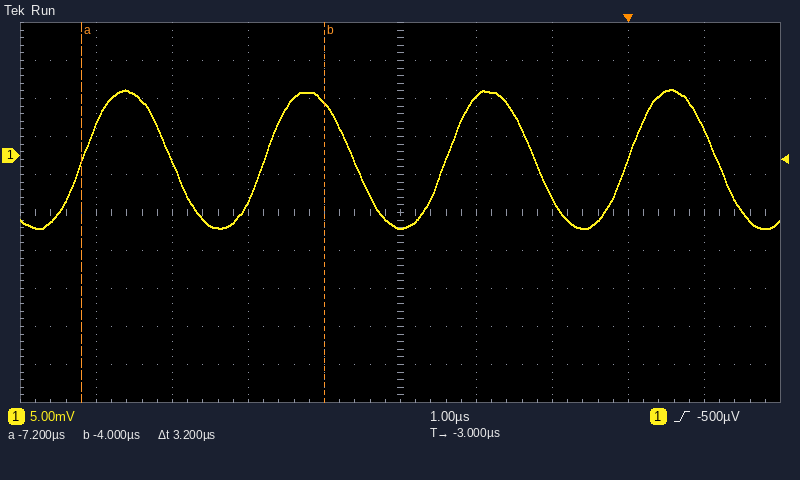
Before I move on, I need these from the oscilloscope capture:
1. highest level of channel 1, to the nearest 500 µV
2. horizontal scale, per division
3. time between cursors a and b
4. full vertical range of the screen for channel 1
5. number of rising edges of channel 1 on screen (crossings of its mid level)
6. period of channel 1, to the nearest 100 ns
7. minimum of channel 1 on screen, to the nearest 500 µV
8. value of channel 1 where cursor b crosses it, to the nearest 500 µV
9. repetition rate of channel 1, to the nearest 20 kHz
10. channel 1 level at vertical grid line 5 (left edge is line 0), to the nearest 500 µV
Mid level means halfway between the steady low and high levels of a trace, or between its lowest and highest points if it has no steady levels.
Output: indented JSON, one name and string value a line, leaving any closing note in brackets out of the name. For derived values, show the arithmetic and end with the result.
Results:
{
  "highest level of channel 1, to the nearest 500 µV": "8.5 mV",
  "horizontal scale, per division": "1 µs",
  "time between cursors a and b": "3.2 µs",
  "full vertical range of the screen for channel 1": "50 mV",
  "number of rising edges of channel 1 on screen": "4",
  "period of channel 1, to the nearest 100 ns": "2.4 µs",
  "minimum of channel 1 on screen, to the nearest 500 µV": "-9.5 mV",
  "value of channel 1 where cursor b crosses it, to the nearest 500 µV": "7.0 mV",
  "repetition rate of channel 1, to the nearest 20 kHz": "1 / 2.4 µs ≈ 417 kHz, so 420 kHz to the nearest 20 kHz",
  "channel 1 level at vertical grid line 5 (left edge is line 0), to the nearest 500 µV": "-9.5 mV"
}
